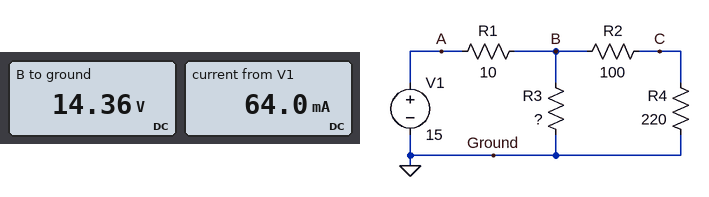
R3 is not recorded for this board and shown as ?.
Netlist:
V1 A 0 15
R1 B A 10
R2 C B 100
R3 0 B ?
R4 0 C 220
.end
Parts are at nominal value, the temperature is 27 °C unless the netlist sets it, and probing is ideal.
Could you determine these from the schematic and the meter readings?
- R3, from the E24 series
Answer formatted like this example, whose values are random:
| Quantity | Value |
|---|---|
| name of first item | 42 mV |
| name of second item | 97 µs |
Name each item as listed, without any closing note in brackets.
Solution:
| Quantity | Value |
|---|---|
| R3, from the E24 series | 750 Ω |
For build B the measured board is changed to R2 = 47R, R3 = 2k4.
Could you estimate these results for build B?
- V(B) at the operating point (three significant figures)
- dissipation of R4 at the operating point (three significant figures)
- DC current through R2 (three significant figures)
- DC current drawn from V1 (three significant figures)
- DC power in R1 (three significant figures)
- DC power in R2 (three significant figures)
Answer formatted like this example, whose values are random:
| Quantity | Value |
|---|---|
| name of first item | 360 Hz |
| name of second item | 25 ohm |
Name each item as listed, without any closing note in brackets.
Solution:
| Quantity | Value |
|---|---|
| V(B) at the operating point | 14.4 V |
| dissipation of R4 at the operating point | 640 mW |
| DC current through R2 | 53.9 mA |
| DC current drawn from V1 | 59.9 mA |
| DC power in R1 | 35.9 mW |
| DC power in R2 | 137 mW |
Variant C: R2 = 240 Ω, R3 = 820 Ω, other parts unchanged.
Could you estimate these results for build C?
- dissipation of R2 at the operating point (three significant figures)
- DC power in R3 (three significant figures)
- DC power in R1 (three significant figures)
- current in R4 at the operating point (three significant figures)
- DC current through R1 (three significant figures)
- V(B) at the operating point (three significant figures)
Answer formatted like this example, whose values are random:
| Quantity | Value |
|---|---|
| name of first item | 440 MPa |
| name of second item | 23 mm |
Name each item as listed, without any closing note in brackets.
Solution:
| Quantity | Value |
|---|---|
| dissipation of R2 at the operating point | 239 mW |
| DC power in R3 | 257 mW |
| DC power in R1 | 24.2 mW |
| current in R4 at the operating point | 31.5 mA |
| DC current through R1 | 49.2 mA |
| V(B) at the operating point | 14.5 V |
